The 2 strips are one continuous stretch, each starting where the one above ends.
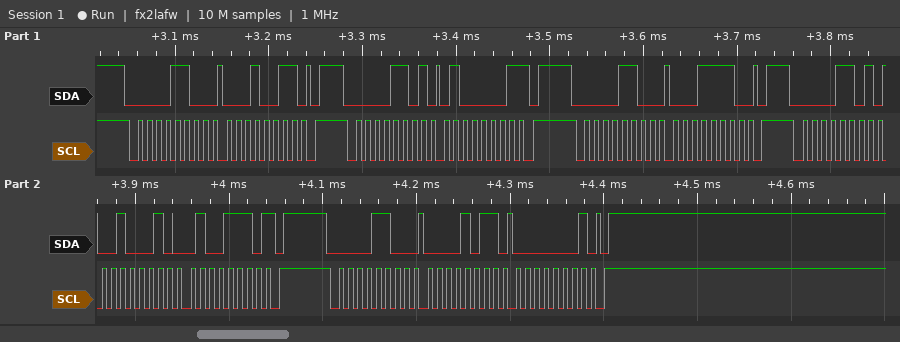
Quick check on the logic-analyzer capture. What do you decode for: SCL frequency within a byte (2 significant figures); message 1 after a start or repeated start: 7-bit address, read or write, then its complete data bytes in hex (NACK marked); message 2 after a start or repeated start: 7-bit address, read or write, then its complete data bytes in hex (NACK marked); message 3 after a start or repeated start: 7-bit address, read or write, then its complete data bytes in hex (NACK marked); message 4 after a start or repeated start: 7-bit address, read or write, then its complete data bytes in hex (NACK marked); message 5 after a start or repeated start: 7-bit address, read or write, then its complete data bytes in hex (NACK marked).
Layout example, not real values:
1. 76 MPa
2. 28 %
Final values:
1. 100 kHz
2. 0x06 write: 13
3. 0x06 read: 41 NACK
4. 0x06 write: 1E
5. 0x06 read: 22 4E NACK
6. 0x06 write: 0B 01
